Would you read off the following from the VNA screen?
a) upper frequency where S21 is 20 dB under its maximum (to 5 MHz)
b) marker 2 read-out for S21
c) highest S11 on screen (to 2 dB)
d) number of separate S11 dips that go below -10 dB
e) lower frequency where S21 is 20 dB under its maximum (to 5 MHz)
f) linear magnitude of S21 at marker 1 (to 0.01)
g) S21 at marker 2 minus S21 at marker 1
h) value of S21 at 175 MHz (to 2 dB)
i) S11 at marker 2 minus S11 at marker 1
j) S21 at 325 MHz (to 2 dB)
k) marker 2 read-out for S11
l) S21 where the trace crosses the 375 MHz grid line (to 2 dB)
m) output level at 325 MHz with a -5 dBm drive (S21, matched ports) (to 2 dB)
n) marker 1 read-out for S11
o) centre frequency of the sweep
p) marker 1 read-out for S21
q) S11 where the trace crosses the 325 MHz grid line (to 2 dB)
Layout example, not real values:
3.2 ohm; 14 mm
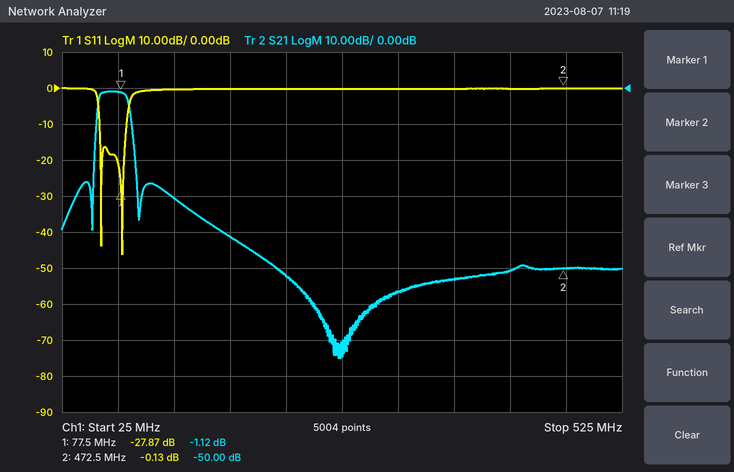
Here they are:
90 MHz; -50.00 dB; 0 dB; 2; 55 MHz; 0.88; -48.88 dB; -42 dB; 27.74 dB; -56 dB; -0.13 dB; -54 dB; -62 dBm; -27.87 dB; 275 MHz; -1.12 dB; 0 dB
